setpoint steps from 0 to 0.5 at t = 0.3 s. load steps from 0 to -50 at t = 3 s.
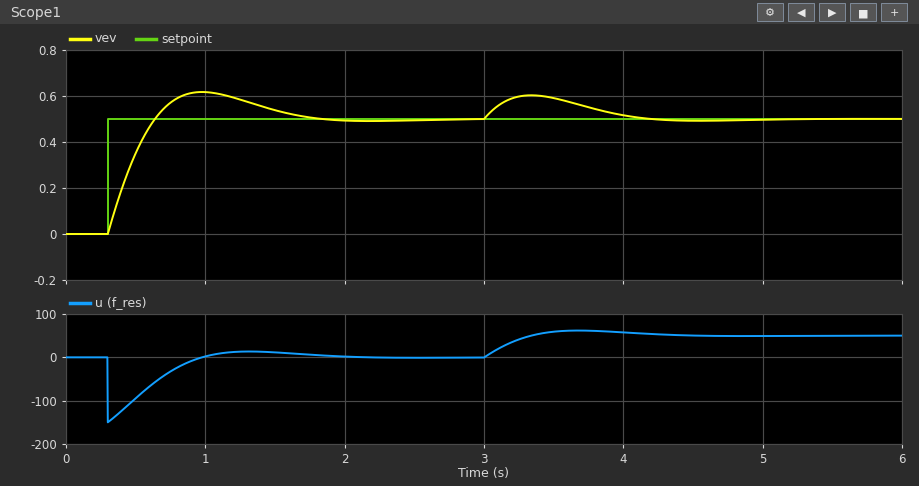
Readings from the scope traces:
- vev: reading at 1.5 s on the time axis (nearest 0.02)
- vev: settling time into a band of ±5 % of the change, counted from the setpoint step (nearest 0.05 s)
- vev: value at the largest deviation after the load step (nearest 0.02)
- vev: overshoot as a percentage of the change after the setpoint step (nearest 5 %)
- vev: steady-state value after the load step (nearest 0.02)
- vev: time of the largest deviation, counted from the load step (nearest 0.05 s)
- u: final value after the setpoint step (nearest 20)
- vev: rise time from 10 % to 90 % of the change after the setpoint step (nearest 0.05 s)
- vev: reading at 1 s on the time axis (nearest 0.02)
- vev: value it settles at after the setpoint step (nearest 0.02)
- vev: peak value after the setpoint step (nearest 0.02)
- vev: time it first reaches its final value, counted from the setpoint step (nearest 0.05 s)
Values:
0.54
1.30 s
0.60
25 %
0.50
0.35 s
0
0.25 s
0.62
0.50
0.62
0.35 s
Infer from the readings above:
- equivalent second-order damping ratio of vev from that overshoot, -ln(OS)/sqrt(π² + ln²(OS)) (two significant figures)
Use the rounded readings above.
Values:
0.40
